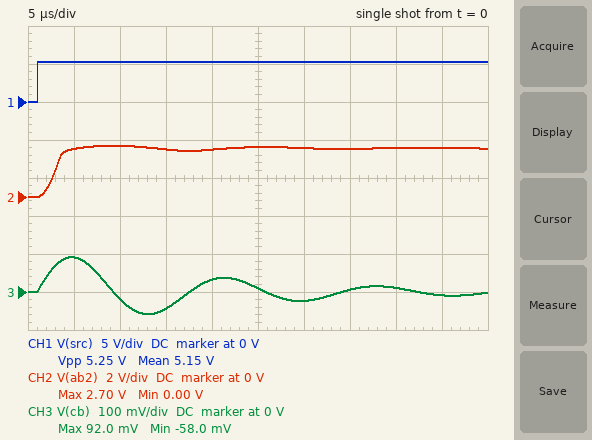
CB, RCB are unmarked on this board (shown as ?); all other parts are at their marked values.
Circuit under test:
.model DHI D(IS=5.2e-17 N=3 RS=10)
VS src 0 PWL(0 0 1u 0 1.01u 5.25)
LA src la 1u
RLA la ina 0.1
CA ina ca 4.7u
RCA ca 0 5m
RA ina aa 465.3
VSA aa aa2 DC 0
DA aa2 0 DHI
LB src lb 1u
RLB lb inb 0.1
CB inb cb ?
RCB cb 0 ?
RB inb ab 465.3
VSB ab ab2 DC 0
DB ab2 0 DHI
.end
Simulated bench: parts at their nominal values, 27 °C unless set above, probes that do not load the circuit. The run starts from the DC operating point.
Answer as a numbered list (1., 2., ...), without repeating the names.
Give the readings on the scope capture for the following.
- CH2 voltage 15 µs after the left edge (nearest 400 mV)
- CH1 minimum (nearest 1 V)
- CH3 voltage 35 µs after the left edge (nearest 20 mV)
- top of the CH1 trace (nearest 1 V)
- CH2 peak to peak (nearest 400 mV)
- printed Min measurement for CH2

1. 2.4 V
2. 0 V
3. 0 V
4. 5 V
5. 2.8 V
6. 0.00 V
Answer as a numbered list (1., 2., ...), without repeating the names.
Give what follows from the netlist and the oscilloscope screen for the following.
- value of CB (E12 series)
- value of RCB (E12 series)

1. 6.8 µF
2. 8.2 mΩ
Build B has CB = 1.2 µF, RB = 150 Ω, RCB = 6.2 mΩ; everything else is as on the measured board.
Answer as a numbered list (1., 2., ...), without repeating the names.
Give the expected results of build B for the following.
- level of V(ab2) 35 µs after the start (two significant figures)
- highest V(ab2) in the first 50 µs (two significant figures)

1. 2.7 V
2. 3.1 V
